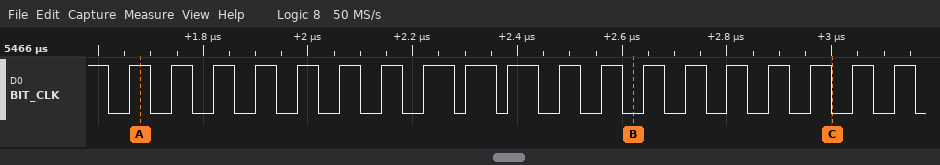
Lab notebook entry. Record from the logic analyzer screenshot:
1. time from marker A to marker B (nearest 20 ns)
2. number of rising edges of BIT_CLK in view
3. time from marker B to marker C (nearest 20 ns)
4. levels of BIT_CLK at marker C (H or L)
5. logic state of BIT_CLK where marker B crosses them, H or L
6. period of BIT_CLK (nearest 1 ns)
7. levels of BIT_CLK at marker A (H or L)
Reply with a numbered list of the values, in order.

1. 940 ns
2. 19
3. 380 ns
4. BIT_CLK=L
5. BIT_CLK=L
6. 81 ns
7. BIT_CLK=H
